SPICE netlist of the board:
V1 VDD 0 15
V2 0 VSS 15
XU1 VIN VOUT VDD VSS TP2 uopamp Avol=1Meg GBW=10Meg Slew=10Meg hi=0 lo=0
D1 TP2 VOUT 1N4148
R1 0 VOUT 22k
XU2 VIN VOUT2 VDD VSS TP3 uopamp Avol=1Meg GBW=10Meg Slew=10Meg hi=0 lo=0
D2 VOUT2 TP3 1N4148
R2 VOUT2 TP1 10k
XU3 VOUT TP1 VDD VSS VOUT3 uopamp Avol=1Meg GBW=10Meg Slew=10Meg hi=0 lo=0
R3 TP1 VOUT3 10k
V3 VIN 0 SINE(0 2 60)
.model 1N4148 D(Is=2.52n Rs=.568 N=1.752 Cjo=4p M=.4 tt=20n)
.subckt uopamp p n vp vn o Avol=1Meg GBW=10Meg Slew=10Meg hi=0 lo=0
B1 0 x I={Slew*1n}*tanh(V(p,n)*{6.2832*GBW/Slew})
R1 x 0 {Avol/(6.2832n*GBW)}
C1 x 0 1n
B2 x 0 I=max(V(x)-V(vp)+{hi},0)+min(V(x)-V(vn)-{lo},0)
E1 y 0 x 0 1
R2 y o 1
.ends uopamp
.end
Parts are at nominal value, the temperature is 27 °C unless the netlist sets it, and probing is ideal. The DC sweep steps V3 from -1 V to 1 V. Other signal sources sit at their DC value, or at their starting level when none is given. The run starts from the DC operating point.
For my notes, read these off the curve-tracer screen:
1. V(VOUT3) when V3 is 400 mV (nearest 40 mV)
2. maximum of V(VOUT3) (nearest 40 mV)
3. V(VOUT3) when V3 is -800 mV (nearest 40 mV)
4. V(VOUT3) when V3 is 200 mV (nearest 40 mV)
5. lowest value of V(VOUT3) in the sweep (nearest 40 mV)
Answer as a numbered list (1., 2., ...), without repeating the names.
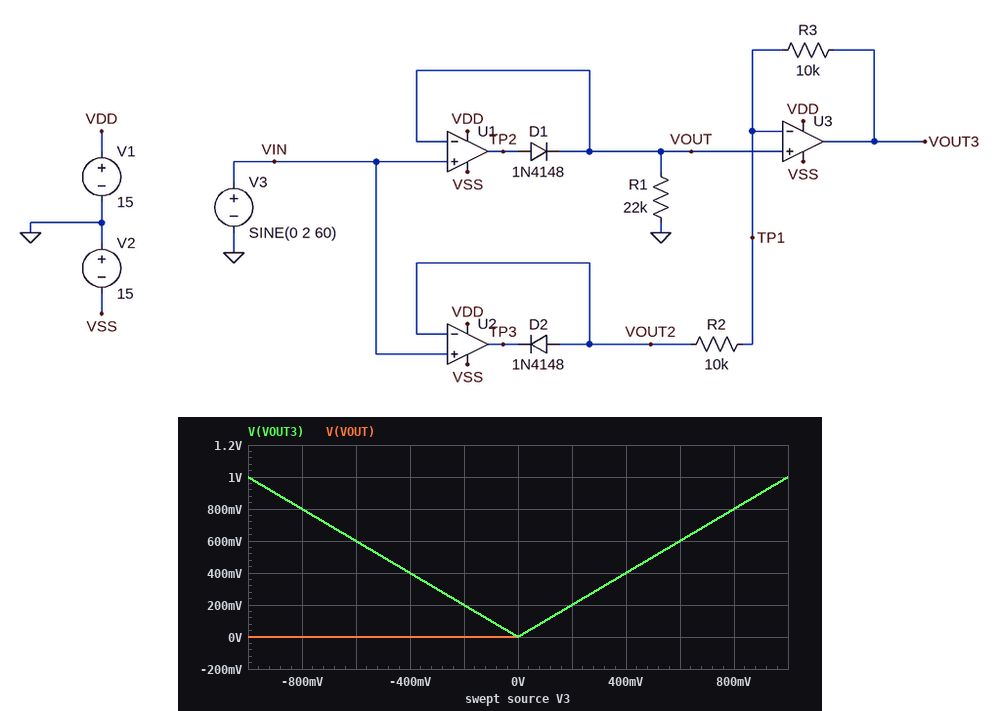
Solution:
1. 400 mV
2. 1.00 V
3. 800 mV
4. 200 mV
5. 0 V
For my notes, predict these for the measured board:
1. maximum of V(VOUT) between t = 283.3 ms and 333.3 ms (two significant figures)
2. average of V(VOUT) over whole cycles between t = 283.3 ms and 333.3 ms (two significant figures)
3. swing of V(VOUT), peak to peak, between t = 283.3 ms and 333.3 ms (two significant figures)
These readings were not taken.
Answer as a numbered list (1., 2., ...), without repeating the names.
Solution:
1. 2.0 V
2. 640 mV
3. 2.0 V
